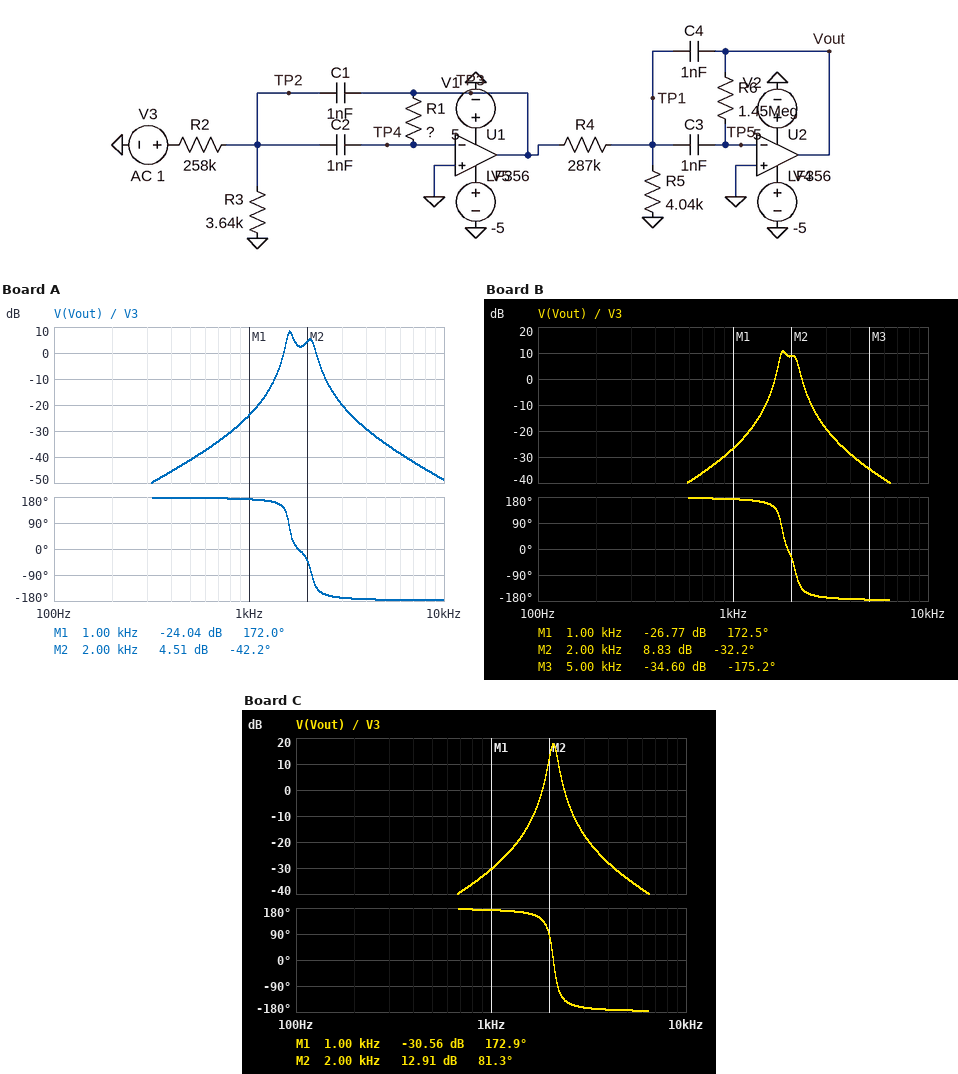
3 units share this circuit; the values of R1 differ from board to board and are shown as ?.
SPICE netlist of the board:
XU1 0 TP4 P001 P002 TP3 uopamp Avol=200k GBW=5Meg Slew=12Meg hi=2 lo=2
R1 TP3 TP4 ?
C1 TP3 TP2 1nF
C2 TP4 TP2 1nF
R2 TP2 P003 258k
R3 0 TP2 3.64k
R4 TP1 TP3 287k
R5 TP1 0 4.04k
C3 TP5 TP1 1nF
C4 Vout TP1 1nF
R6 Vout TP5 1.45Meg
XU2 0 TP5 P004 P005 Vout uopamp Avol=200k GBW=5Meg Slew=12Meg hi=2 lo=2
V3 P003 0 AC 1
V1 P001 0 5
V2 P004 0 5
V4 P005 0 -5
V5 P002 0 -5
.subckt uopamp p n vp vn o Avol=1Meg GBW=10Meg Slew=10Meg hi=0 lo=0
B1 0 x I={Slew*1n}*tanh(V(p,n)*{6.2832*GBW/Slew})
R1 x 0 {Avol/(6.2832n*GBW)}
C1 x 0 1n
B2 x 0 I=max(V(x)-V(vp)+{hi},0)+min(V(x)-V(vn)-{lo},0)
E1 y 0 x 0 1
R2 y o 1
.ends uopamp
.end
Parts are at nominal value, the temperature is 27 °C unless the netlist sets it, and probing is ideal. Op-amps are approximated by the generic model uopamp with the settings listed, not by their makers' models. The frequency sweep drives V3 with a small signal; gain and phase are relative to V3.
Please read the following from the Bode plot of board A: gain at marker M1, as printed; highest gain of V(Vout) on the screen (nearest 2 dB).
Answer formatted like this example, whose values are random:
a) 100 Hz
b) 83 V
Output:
a) -24.04 dB
b) 8 dB
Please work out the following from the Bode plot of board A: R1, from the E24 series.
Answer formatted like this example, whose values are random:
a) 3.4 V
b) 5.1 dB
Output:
a) 2.7 MΩ
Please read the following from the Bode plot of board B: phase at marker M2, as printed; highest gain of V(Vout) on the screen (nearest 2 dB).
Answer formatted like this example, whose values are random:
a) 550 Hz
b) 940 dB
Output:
a) -32.2 deg
b) 10 dB
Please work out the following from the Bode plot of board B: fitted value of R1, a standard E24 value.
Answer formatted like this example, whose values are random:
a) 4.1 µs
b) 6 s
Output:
a) 2.2 MΩ
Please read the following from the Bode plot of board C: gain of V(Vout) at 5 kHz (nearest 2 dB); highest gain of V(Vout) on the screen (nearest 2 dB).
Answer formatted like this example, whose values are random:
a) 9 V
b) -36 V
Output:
a) -34 dB
b) 18 dB
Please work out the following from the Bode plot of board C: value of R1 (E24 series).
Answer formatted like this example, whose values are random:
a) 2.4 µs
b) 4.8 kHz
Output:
a) 1.6 MΩ
